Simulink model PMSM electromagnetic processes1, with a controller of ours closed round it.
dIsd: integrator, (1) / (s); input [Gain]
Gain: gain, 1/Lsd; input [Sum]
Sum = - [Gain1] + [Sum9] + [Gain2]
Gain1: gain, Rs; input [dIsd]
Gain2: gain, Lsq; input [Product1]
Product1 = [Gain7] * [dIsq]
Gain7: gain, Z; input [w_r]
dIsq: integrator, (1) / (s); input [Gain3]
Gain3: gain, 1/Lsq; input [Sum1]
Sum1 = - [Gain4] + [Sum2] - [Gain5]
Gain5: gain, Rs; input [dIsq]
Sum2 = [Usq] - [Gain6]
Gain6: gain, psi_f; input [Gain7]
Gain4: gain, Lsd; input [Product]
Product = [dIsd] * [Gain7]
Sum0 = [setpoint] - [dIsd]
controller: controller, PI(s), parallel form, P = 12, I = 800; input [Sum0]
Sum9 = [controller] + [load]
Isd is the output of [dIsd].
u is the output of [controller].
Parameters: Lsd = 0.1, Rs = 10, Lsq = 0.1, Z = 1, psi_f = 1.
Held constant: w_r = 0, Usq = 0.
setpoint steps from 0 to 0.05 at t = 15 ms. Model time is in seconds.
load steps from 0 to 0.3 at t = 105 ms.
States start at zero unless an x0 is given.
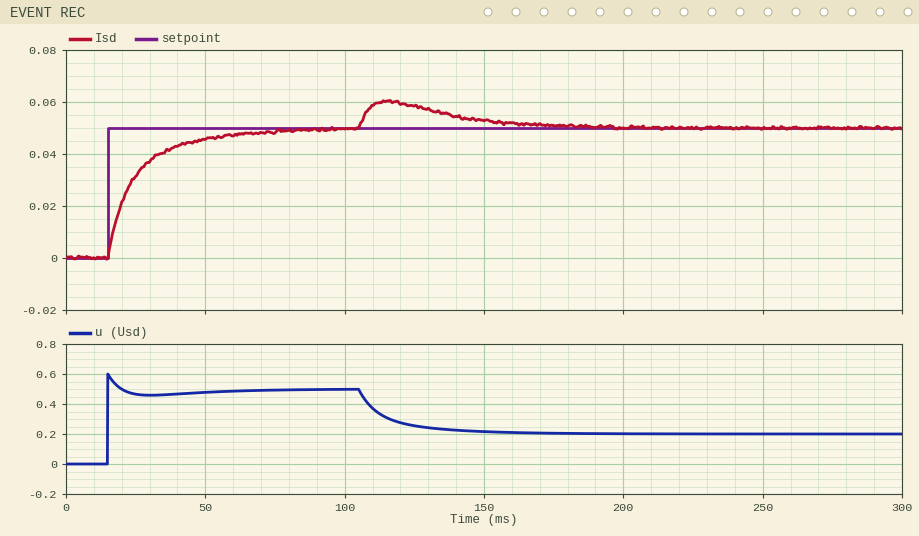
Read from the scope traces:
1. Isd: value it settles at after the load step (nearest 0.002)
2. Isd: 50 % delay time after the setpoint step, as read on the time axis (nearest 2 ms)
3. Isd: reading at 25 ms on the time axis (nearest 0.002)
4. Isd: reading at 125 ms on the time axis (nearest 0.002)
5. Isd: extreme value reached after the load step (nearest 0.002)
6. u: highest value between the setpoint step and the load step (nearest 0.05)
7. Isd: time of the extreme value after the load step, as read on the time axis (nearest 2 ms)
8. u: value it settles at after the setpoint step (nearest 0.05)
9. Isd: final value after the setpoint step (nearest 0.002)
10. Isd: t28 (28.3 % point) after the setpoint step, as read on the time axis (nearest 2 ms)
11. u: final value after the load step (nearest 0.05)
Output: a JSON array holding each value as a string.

["0.050", "22 ms", "0.032", "0.058", "0.060", "0.60", "116 ms", "0.50", "0.050", "18 ms", "0.20"]
